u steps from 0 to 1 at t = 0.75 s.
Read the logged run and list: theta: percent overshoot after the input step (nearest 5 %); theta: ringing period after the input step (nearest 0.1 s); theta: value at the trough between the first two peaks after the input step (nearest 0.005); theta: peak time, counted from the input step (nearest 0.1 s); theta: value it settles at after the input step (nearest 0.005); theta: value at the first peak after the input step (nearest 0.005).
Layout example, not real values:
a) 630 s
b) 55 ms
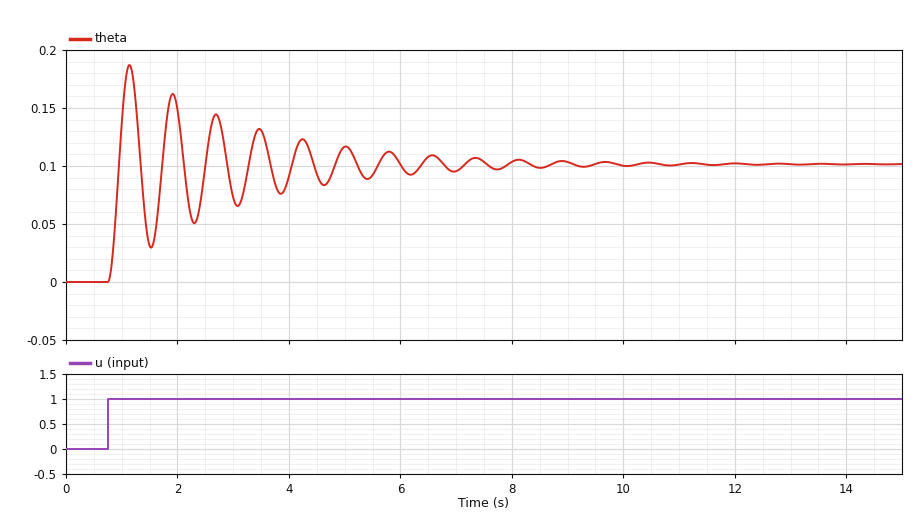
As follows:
a) 85 %
b) 0.8 s
c) 0.030
d) 0.4 s
e) 0.100
f) 0.185
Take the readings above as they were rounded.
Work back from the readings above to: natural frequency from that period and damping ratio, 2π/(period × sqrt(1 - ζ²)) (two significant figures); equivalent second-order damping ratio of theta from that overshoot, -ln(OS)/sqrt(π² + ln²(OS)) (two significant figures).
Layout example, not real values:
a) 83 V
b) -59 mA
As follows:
a) 7.9 rad/s
b) 0.052
